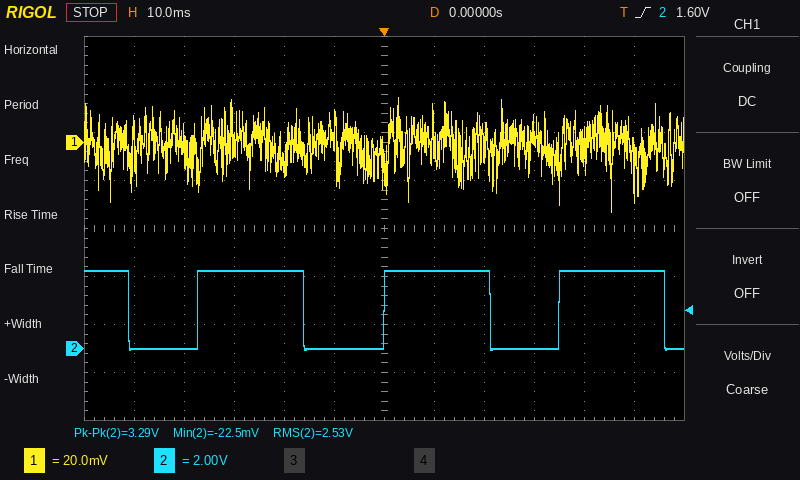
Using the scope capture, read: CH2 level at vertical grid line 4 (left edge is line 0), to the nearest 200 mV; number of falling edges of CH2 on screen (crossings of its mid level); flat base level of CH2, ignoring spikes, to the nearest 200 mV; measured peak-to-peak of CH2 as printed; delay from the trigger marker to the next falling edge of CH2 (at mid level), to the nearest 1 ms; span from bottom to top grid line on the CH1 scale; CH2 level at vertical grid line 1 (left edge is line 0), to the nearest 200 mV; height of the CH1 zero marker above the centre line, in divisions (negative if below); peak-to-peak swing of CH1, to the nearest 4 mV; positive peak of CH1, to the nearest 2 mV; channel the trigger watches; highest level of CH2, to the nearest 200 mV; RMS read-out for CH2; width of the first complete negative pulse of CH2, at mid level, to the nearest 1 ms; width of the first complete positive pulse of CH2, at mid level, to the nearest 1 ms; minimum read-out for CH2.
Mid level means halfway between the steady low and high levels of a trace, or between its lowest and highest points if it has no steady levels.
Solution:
3.2 V
4
0.0 V
3.29 V
21 ms
160 mV
0.0 V
+1.8 div
48 mV
18 mV
CH2
3.2 V
2.53 V
14 ms
21 ms
-22.5 mV
